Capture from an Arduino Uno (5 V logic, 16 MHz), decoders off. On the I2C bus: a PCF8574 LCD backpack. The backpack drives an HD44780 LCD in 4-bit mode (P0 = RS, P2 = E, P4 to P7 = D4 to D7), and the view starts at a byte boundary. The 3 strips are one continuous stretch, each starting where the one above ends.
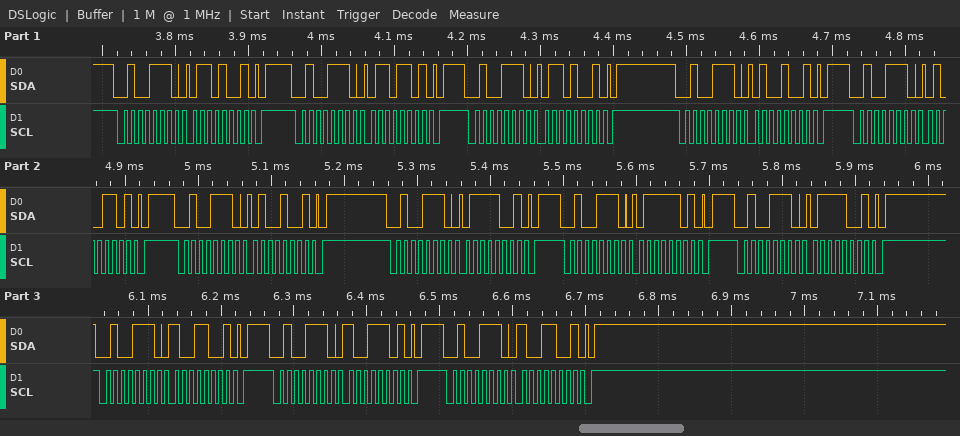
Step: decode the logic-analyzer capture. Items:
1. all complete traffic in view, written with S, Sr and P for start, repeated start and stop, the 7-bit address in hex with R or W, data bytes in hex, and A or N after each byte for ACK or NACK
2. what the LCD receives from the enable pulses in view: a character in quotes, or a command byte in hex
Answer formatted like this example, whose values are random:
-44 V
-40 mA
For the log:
S 27W A 69 A P S 27W A 6D A P S 27W A 69 A P S 27W A 49 A P S 27W A 4D A P S 27W A 49 A P S 27W A 79 A P S 27W A 7D A P S 27W A 79 A P S 27W A 99 A P S 27W A 9D A P S 27W A 99 A P
'd' 'y'
